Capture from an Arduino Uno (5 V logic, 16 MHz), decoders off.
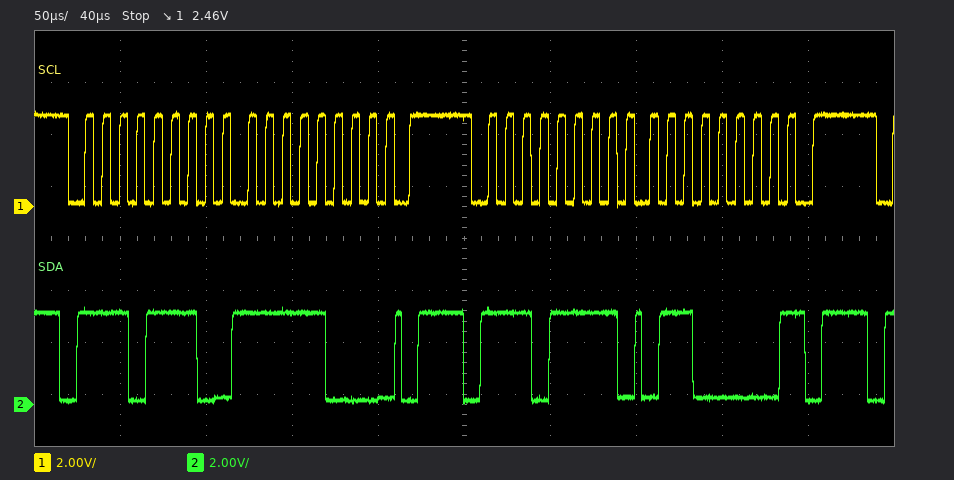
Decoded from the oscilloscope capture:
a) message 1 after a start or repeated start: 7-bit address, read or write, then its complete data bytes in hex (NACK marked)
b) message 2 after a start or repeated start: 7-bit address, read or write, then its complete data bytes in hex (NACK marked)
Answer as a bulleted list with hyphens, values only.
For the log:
- 0x77 write: F8
- 0x77 read: 60 NACK
